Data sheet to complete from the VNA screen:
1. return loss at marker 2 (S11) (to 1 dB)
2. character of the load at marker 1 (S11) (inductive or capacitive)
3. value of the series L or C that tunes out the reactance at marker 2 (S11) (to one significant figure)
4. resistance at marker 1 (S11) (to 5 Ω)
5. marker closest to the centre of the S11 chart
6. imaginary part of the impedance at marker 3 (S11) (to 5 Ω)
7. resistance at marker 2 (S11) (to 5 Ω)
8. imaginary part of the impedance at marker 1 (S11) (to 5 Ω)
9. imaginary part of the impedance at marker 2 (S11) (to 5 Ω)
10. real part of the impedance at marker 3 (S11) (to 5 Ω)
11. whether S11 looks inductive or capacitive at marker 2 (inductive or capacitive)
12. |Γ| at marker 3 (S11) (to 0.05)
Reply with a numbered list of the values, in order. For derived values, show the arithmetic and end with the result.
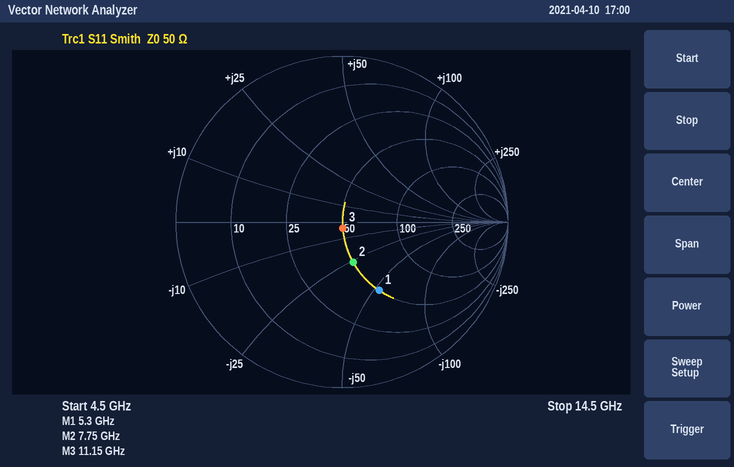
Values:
1. 12 dB
2. capacitive
3. L = 25 Ω/(2π × 7.75 GHz) ≈ 513 pH, so 500 pH to one significant figure
4. 50 Ω
5. marker 3
6. -5 Ω
7. 50 Ω
8. -55 Ω
9. -25 Ω
10. 50 Ω
11. capacitive
12. 0.05
